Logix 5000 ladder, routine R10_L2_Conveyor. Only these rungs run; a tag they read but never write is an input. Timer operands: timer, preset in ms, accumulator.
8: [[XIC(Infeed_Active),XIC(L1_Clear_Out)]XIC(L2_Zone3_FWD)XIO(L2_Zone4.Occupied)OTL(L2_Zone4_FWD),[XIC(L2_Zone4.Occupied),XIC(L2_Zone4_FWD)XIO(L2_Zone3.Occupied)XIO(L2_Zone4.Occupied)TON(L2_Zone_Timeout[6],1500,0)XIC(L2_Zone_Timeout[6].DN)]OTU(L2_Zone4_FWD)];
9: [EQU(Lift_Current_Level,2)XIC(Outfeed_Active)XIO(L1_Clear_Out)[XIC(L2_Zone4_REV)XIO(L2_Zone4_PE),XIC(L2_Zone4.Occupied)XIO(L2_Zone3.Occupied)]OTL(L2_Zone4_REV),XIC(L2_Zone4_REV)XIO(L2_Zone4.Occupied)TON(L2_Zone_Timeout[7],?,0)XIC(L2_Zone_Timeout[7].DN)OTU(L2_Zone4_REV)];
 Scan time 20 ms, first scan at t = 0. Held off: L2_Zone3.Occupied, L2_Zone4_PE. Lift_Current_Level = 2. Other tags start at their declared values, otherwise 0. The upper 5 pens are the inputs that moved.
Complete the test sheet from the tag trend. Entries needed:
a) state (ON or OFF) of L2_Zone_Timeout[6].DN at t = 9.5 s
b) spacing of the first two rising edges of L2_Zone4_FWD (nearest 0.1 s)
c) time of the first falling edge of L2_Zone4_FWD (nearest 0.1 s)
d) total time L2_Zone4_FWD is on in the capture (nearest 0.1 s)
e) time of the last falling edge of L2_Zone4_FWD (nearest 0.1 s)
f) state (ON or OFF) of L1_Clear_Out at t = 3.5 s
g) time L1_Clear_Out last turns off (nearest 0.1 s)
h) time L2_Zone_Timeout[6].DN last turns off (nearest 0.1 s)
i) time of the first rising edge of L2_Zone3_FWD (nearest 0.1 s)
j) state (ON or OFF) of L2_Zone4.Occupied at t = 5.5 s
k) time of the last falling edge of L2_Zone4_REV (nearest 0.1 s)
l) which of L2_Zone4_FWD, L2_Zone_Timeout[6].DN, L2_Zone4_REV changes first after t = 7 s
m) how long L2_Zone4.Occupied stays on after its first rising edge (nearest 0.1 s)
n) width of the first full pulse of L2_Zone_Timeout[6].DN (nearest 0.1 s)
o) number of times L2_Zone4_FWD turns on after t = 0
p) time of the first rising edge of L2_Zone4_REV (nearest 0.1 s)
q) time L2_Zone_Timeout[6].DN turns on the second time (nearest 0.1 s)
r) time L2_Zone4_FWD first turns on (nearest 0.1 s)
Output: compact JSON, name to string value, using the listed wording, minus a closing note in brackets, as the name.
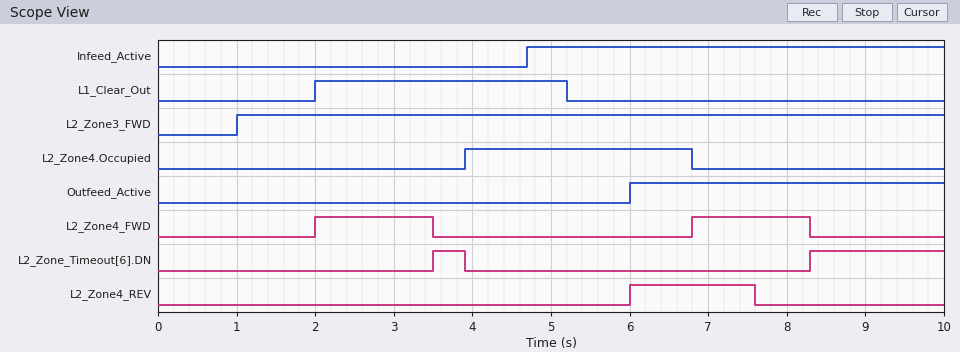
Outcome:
{"state (ON or OFF) of L2_Zone_Timeout[6].DN at t = 9.5 s": "ON", "spacing of the first two rising edges of L2_Zone4_FWD": "4.8 s", "time of the first falling edge of L2_Zone4_FWD": "3.5 s", "total time L2_Zone4_FWD is on in the capture": "3.0 s", "time of the last falling edge of L2_Zone4_FWD": "8.3 s", "state (ON or OFF) of L1_Clear_Out at t = 3.5 s": "ON", "time L1_Clear_Out last turns off": "5.2 s", "time L2_Zone_Timeout[6].DN last turns off": "3.9 s", "time of the first rising edge of L2_Zone3_FWD": "1.0 s", "state (ON or OFF) of L2_Zone4.Occupied at t = 5.5 s": "ON", "time of the last falling edge of L2_Zone4_REV": "7.6 s", "which of L2_Zone4_FWD, L2_Zone_Timeout[6].DN, L2_Zone4_REV changes first after t = 7 s": "L2_Zone4_REV", "how long L2_Zone4.Occupied stays on after its first rising edge": "2.9 s", "width of the first full pulse of L2_Zone_Timeout[6].DN": "0.4 s", "number of times L2_Zone4_FWD turns on after t = 0": "2", "time of the first rising edge of L2_Zone4_REV": "6.0 s", "time L2_Zone_Timeout[6].DN turns on the second time": "8.3 s", "time L2_Zone4_FWD first turns on": "2.0 s"}
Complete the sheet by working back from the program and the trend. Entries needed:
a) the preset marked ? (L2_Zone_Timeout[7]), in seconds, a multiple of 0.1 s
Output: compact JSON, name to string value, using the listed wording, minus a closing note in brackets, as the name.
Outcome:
{"the preset marked ? (L2_Zone_Timeout[7]), in seconds, a multiple of 0.1 s": "0.8 s"}
